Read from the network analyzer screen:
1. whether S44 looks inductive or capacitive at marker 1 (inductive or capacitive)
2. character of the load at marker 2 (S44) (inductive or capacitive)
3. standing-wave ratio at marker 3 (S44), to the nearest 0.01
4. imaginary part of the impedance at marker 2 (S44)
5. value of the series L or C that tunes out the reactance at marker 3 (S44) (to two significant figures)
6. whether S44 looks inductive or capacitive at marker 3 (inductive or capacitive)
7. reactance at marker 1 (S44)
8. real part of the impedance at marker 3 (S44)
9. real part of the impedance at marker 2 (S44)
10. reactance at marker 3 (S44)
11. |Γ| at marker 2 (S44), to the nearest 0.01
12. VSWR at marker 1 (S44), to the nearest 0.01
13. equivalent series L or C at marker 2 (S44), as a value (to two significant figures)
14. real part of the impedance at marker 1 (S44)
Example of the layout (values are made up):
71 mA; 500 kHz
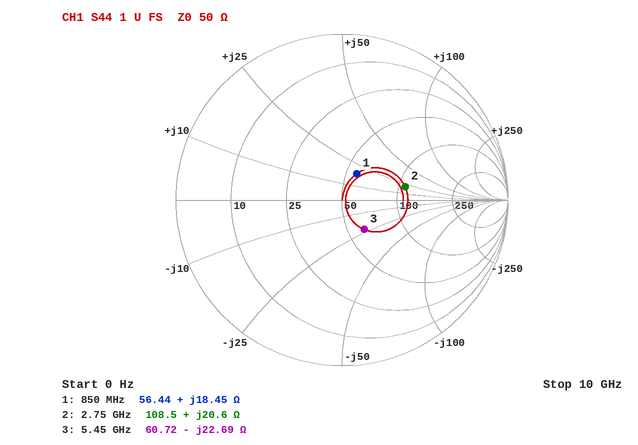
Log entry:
inductive; inductive; 1.57; +20.6 Ω; 660 pH; capacitive; +18.45 Ω; 60.72 Ω; 108.5 Ω; -22.69 Ω; 0.39; 1.44; 1.2 nH; 56.44 Ω
